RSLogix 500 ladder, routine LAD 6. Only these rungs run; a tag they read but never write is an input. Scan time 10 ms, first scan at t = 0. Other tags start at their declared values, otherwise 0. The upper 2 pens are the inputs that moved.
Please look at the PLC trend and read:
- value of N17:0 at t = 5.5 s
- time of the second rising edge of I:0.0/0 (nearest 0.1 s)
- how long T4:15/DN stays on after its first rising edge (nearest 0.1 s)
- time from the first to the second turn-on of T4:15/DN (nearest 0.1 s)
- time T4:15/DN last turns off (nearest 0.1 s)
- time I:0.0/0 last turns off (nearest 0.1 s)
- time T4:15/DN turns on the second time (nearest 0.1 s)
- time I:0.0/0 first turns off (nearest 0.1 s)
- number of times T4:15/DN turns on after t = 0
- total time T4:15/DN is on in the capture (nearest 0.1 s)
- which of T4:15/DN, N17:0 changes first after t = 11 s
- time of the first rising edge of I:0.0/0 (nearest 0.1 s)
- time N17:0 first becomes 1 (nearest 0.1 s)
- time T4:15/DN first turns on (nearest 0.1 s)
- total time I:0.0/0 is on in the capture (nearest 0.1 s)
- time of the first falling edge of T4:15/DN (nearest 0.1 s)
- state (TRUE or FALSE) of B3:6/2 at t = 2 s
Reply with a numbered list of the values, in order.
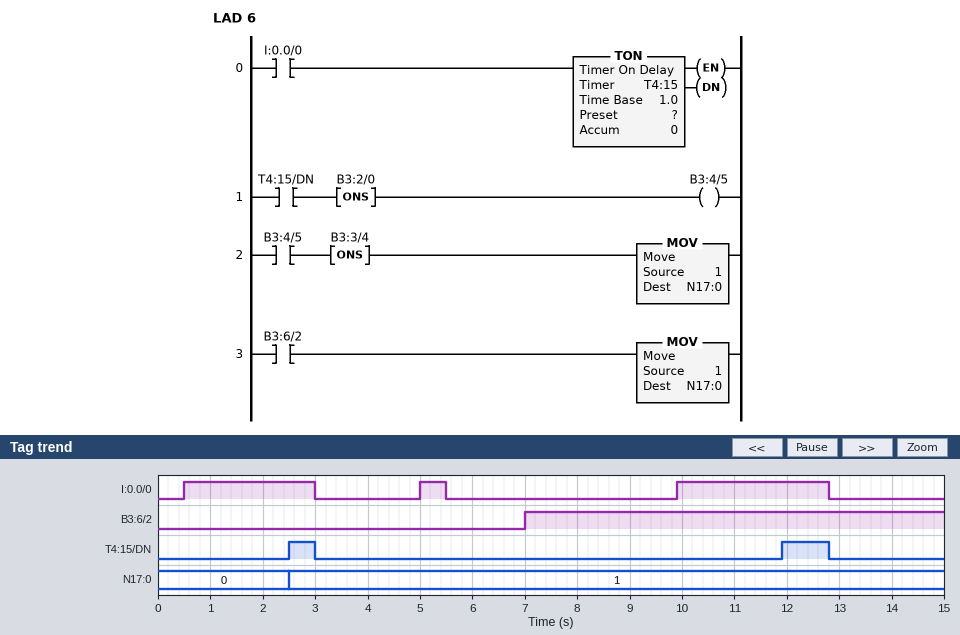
1. 1
2. 5.0 s
3. 0.5 s
4. 9.4 s
5. 12.8 s
6. 12.8 s
7. 11.9 s
8. 3.0 s
9. 2
10. 1.4 s
11. T4:15/DN
12. 0.5 s
13. 2.5 s
14. 2.5 s
15. 5.9 s
16. 3.0 s
17. FALSE
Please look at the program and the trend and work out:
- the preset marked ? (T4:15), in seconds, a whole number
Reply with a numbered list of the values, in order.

1. 2 s
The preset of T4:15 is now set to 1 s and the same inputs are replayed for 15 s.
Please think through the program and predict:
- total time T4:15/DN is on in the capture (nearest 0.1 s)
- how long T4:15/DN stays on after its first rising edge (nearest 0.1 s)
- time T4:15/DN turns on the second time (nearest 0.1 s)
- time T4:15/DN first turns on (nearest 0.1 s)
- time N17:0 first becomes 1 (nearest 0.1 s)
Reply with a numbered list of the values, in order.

1. 3.4 s
2. 1.5 s
3. 10.9 s
4. 1.5 s
5. 1.5 s
